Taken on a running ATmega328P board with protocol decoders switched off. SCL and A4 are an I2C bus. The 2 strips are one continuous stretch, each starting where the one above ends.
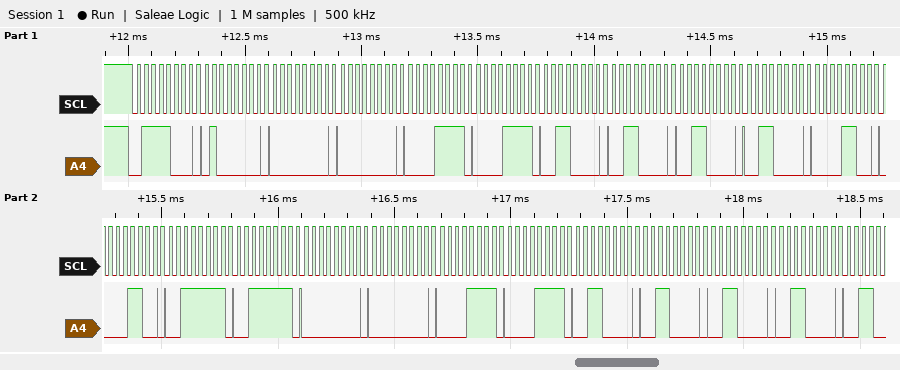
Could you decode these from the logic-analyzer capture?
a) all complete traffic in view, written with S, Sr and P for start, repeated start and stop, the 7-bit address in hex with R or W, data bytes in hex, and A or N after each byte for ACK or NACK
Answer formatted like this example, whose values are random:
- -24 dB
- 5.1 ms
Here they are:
- S 3CW A 40 A 00 A 00 A 0F A 0F A 30 A 30 A 30 A 30 A 0C A 0C A 3F A 3F A 00 A 00 A 0F A 0F A 30 A 30 A 30 A 30 A
